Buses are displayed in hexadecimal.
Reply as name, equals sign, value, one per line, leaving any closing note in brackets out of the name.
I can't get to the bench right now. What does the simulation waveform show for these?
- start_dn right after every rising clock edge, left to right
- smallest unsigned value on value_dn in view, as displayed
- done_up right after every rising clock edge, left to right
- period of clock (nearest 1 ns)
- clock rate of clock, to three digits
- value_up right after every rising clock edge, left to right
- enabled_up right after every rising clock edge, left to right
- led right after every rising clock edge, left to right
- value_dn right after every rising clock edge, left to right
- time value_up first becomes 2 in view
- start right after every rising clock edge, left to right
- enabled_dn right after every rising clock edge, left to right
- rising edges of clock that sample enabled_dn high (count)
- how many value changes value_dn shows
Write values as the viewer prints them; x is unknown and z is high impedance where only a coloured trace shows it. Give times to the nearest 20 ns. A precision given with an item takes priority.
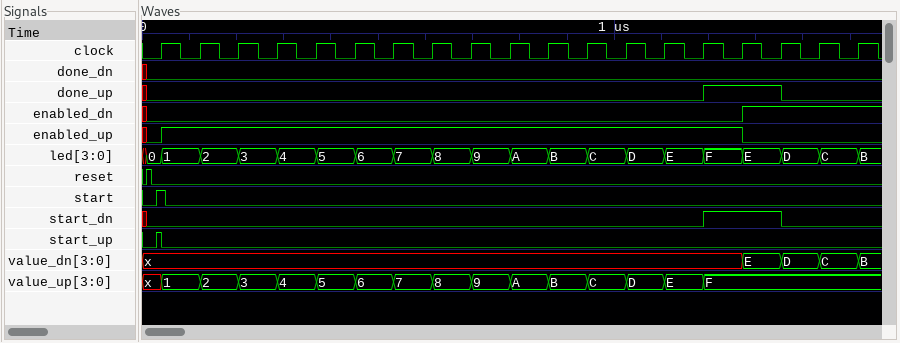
start_dn right after every rising clock edge, left to right = 0 0 0 0 0 0 0 0 0 0 0 0 0 0 1 1 0 0 0
smallest unsigned value on value_dn in view, as displayed = B
done_up right after every rising clock edge, left to right = 0 0 0 0 0 0 0 0 0 0 0 0 0 0 1 1 0 0 0
period of clock = 82 ns
clock rate of clock, to three digits = 12.2 MHz
value_up right after every rising clock edge, left to right = 1, 2, 3, 4, 5, 6, 7, 8, 9, A, B, C, D, E, F, F, F, F, F
enabled_up right after every rising clock edge, left to right = 1 1 1 1 1 1 1 1 1 1 1 1 1 1 1 0 0 0 0
led right after every rising clock edge, left to right = 1, 2, 3, 4, 5, 6, 7, 8, 9, A, B, C, D, E, F, E, D, C, B
value_dn right after every rising clock edge, left to right = x, x, x, x, x, x, x, x, x, x, x, x, x, x, x, E, D, C, B
time value_up first becomes 2 in view = 120 ns
start right after every rising clock edge, left to right = 1 0 0 0 0 0 0 0 0 0 0 0 0 0 0 0 0 0 0
enabled_dn right after every rising clock edge, left to right = 0 0 0 0 0 0 0 0 0 0 0 0 0 0 0 1 1 1 1
rising edges of clock that sample enabled_dn high = 3
how many value changes value_dn shows = 4
